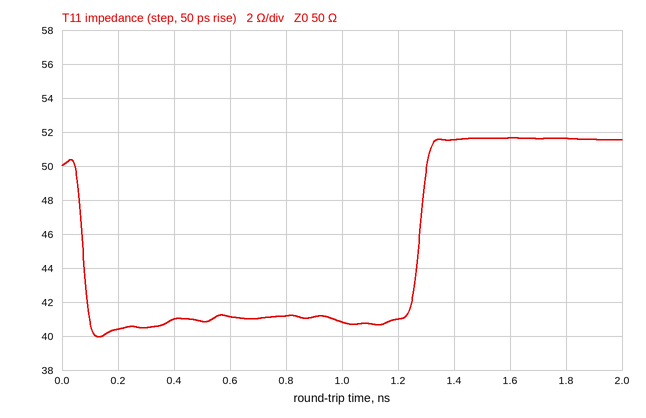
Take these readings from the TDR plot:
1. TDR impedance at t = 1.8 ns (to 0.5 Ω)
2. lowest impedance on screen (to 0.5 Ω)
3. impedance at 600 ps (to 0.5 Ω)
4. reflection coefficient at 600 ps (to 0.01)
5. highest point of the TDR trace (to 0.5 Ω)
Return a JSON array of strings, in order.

["51.5 Ω", "40.0 Ω", "41.0 Ω", "-0.10", "51.5 Ω"]
